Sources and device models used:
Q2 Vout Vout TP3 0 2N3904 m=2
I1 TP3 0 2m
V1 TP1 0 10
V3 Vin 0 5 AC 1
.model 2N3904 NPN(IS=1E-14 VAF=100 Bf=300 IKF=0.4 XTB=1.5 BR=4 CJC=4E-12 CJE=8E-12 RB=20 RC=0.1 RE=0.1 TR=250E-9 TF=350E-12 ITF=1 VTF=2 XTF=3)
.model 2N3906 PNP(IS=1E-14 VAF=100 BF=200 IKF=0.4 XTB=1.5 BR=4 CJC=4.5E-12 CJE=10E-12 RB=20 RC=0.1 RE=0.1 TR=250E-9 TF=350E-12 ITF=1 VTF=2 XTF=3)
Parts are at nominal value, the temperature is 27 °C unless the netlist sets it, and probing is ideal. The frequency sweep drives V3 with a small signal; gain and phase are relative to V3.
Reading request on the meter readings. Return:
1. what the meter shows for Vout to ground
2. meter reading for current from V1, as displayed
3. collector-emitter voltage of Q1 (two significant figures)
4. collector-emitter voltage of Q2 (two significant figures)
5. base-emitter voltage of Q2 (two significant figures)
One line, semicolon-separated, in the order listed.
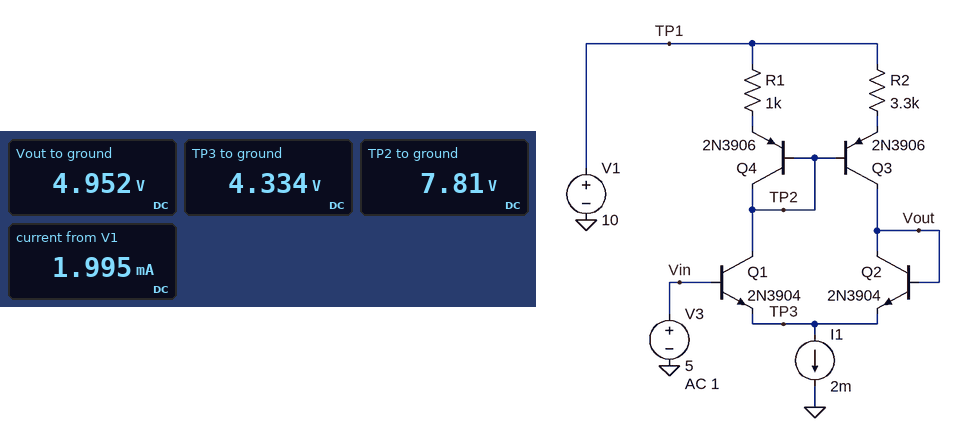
4.952 V; 1.995 mA; 3.5 V; 620 mV; 620 mV
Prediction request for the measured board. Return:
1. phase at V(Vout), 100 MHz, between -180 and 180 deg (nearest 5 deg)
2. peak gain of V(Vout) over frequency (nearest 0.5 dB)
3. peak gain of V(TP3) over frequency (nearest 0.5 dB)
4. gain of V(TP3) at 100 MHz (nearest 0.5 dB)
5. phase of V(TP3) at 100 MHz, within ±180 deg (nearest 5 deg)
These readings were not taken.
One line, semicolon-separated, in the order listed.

0 deg; 0 dB; 0 dB; -0.5 dB; 0 deg
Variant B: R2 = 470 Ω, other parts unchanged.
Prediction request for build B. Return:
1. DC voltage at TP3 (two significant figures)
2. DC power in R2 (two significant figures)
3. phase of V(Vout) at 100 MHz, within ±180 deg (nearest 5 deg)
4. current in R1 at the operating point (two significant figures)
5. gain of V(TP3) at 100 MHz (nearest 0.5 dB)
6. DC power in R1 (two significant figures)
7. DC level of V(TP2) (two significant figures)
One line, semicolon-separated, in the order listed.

4.4 V; 850 µW; -5 deg; 650 µA; -1.0 dB; 420 µW; 8.7 V
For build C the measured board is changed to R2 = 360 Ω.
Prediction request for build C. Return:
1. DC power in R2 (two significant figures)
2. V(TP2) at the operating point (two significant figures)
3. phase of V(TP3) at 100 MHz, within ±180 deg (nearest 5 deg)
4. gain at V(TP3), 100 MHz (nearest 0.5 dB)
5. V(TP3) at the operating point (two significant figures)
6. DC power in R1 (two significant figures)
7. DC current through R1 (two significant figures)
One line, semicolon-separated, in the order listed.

760 µW; 8.8 V; -5 deg; -1.5 dB; 4.4 V; 300 µW; 550 µA
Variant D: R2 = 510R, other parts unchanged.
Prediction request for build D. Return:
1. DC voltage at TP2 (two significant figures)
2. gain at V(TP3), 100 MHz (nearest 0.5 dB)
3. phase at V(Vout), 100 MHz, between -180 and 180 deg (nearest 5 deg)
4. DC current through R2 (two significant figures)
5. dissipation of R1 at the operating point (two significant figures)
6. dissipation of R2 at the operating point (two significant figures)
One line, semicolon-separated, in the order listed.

8.7 V; -1.0 dB; -5 deg; 1.3 mA; 470 µW; 880 µW
